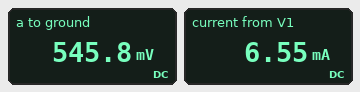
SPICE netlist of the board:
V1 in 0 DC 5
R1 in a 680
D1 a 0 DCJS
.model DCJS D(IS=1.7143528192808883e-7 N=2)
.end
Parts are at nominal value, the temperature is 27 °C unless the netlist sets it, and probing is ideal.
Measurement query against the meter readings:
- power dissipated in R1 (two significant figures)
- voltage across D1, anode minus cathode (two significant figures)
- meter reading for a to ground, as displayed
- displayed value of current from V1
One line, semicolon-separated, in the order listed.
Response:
29 mW; 550 mV; 545.8 mV; 6.55 mA
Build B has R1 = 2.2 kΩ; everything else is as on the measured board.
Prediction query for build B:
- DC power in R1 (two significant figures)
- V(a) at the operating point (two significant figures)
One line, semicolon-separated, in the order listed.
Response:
9.3 mW; 490 mV
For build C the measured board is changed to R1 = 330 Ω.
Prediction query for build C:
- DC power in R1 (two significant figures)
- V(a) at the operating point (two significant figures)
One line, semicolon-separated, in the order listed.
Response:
59 mW; 580 mV
